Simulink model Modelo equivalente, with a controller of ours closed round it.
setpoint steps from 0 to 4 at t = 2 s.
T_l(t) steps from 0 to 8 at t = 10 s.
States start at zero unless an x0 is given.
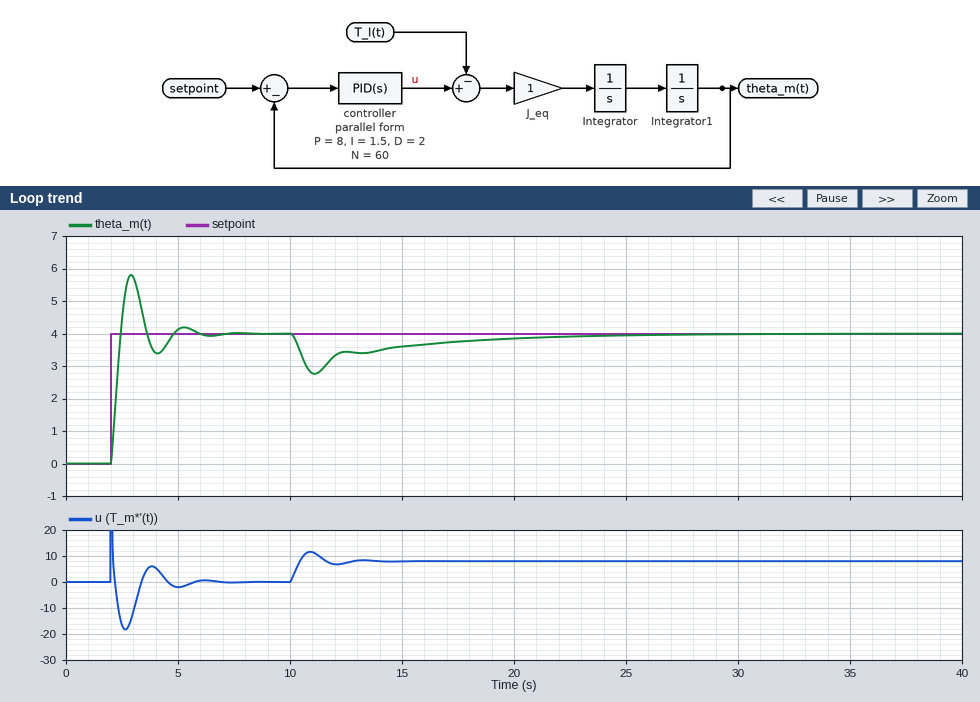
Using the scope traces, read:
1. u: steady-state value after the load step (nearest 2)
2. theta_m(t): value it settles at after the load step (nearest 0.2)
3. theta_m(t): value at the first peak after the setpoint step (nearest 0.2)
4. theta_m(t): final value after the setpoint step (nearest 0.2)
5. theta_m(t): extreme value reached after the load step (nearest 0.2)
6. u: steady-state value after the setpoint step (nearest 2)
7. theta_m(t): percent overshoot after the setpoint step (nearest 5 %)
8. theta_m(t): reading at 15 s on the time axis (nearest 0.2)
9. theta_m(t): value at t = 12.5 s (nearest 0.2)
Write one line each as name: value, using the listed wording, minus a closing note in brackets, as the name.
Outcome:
u: steady-state value after the load step: 8
theta_m(t): value it settles at after the load step: 4.0
theta_m(t): value at the first peak after the setpoint step: 5.8
theta_m(t): final value after the setpoint step: 4.0
theta_m(t): extreme value reached after the load step: 2.8
u: steady-state value after the setpoint step: 0
theta_m(t): percent overshoot after the setpoint step: 45 %
theta_m(t): reading at 15 s on the time axis: 3.6
theta_m(t): value at t = 12.5 s: 3.4
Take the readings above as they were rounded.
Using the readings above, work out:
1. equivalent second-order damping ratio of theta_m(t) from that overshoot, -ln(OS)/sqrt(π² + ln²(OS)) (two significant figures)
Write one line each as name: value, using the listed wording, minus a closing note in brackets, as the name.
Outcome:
equivalent second-order damping ratio of theta_m(t) from that overshoot, -ln(OS)/sqrt(π² + ln²(OS)): 0.25
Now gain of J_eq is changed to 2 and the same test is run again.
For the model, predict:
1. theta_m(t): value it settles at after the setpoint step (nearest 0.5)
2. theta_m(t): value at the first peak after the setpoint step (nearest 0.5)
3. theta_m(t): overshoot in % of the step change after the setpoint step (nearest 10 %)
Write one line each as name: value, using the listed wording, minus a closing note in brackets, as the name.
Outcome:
theta_m(t): value it settles at after the setpoint step: 4.0
theta_m(t): value at the first peak after the setpoint step: 5.5
theta_m(t): overshoot in % of the step change after the setpoint step: 30 %
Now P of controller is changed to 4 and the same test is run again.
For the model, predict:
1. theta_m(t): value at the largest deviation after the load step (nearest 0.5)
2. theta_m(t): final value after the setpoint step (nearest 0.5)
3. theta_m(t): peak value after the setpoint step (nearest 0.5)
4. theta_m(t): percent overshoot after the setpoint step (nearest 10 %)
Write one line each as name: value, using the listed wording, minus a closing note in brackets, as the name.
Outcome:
theta_m(t): value at the largest deviation after the load step: 2.0
theta_m(t): final value after the setpoint step: 4.0
theta_m(t): peak value after the setpoint step: 5.5
theta_m(t): percent overshoot after the setpoint step: 40 %
